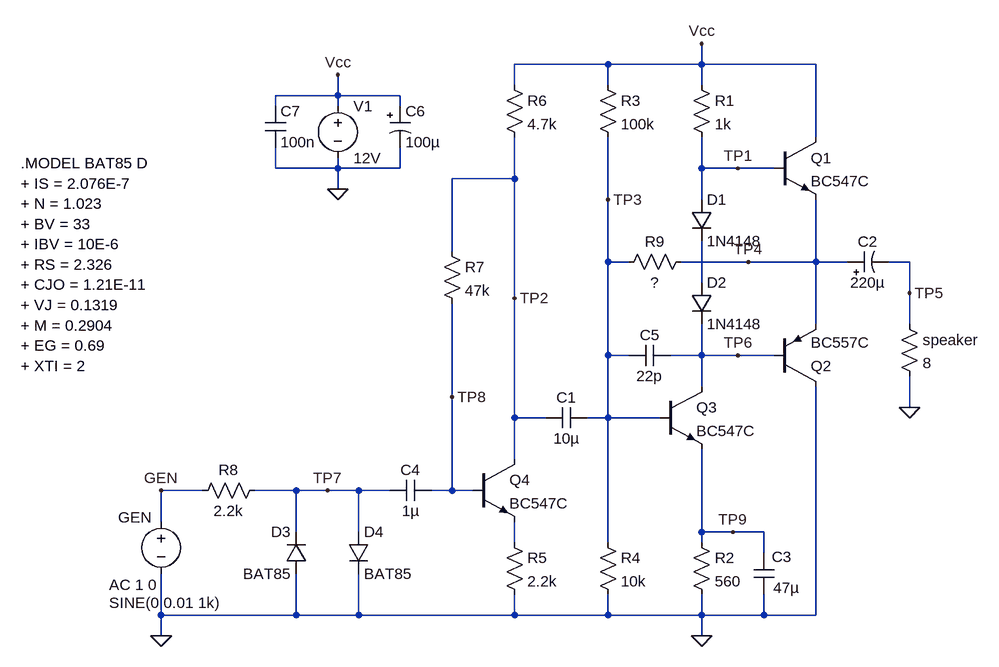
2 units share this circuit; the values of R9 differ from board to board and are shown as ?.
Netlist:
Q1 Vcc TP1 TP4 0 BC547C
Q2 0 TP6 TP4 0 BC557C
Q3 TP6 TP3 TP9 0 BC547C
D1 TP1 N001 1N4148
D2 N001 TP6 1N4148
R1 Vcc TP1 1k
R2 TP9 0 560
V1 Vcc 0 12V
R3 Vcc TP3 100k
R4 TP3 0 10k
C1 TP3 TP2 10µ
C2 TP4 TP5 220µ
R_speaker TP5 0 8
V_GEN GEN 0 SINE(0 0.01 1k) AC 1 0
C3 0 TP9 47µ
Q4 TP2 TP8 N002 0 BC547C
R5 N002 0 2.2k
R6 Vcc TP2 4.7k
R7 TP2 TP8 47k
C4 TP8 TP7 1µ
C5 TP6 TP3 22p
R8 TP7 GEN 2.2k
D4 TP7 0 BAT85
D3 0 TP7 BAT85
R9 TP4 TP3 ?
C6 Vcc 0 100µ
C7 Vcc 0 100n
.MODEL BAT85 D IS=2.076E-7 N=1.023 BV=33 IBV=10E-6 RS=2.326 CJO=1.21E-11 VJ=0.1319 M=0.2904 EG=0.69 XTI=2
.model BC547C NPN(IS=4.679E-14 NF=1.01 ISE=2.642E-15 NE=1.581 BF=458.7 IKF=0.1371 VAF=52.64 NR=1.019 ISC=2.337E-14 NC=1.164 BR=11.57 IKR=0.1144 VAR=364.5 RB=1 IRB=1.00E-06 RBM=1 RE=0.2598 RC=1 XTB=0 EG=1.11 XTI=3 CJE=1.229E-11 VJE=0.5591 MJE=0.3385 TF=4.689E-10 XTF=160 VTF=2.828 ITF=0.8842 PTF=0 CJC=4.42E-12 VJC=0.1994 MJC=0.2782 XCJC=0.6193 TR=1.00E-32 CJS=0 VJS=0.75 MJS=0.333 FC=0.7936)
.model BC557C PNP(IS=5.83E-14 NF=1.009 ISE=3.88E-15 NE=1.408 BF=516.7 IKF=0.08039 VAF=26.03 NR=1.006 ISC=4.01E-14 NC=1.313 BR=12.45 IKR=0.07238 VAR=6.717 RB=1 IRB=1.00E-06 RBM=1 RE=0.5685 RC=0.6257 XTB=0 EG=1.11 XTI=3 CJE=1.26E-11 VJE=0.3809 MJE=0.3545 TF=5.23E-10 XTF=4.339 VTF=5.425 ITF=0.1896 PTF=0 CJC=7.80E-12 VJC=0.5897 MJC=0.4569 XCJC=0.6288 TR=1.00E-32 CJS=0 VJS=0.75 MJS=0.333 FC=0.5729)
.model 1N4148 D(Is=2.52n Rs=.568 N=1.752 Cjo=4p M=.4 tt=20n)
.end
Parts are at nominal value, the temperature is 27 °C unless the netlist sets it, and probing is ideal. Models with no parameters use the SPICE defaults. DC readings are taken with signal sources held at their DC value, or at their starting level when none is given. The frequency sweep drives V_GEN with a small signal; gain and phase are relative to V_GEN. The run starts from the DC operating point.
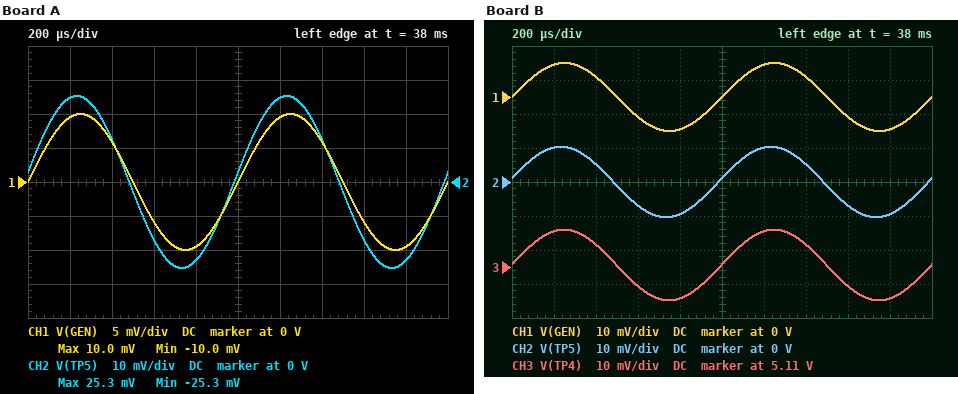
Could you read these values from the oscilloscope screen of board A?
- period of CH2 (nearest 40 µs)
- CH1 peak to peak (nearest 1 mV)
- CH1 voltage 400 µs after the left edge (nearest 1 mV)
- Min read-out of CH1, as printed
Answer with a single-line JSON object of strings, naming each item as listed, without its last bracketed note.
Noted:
{"period of CH2": "1.00 ms", "CH1 peak to peak": "20 mV", "CH1 voltage 400 µs after the left edge": "6 mV", "Min read-out of CH1, as printed": "-10.0 mV"}
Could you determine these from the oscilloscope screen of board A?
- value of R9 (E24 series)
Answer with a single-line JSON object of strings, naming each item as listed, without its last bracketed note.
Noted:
{"value of R9": "6.8 kΩ"}
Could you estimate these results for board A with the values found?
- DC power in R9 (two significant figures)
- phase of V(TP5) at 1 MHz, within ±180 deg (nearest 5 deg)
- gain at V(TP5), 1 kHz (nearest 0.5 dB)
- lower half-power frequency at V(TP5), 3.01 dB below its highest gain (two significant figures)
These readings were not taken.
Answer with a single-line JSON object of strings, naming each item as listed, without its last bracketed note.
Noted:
{"DC power in R9": "630 µW", "phase of V(TP5) at 1 MHz, within ±180 deg": "-80 deg", "gain at V(TP5), 1 kHz": "8.0 dB", "lower half-power frequency at V(TP5), 3.01 dB below its highest gain": "98 Hz"}
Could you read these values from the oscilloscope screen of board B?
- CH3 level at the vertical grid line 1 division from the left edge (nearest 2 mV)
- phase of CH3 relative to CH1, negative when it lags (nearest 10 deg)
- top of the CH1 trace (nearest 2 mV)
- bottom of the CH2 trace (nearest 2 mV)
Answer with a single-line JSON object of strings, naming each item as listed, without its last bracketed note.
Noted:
{"CH3 level at the vertical grid line 1 division from the left edge": "5.120 V", "phase of CH3 relative to CH1, negative when it lags": "0 deg", "top of the CH1 trace": "10 mV", "bottom of the CH2 trace": "-10 mV"}
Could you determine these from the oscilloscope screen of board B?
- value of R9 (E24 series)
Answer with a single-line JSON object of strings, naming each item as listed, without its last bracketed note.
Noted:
{"value of R9": "2.7 kΩ"}
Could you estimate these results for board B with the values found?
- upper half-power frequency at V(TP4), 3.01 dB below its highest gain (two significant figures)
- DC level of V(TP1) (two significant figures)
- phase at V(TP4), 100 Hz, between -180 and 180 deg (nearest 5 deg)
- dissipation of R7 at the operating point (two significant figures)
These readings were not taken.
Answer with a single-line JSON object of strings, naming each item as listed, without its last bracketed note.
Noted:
{"upper half-power frequency at V(TP4), 3.01 dB below its highest gain": "1.4 MHz", "DC level of V(TP1)": "5.8 V", "phase at V(TP4), 100 Hz, between -180 and 180 deg": "10 deg", "dissipation of R7 at the operating point": "600 nW"}
